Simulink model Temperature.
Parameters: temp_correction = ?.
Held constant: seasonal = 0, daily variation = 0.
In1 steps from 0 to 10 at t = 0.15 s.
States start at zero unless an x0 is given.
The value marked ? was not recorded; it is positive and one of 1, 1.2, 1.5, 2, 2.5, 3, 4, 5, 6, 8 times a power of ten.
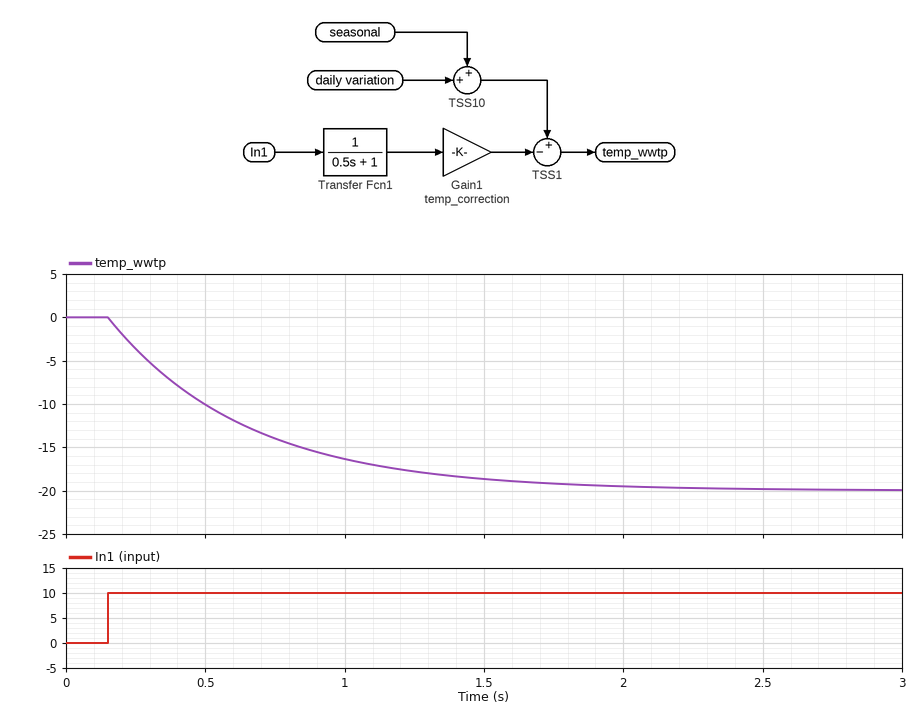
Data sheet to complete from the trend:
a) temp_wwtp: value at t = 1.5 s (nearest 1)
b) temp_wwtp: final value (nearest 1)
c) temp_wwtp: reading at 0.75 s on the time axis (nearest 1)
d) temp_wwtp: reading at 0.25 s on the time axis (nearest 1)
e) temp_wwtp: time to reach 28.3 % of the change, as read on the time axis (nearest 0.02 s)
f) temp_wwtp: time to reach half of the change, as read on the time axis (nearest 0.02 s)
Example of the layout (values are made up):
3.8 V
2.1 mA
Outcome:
-19
-20
-14
-4
0.32 s
0.50 s
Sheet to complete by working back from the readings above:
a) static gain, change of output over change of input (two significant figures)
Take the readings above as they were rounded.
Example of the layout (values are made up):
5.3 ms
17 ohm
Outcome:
-2.0
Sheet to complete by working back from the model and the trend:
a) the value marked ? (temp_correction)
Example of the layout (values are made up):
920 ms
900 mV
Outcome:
2
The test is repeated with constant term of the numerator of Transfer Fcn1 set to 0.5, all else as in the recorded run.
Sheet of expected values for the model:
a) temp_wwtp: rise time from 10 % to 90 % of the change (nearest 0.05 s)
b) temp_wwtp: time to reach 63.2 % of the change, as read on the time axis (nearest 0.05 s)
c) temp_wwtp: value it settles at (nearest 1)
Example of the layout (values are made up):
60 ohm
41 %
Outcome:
1.10 s
0.65 s
-10
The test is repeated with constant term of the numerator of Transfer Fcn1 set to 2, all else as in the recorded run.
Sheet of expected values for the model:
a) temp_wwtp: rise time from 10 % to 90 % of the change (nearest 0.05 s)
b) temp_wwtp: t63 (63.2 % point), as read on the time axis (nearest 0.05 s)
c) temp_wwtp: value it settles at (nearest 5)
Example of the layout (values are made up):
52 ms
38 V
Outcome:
1.10 s
0.65 s
-40
